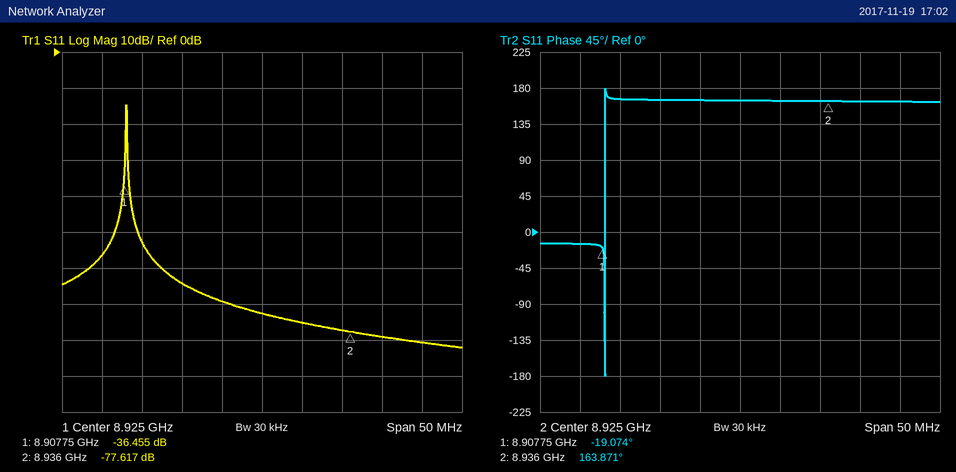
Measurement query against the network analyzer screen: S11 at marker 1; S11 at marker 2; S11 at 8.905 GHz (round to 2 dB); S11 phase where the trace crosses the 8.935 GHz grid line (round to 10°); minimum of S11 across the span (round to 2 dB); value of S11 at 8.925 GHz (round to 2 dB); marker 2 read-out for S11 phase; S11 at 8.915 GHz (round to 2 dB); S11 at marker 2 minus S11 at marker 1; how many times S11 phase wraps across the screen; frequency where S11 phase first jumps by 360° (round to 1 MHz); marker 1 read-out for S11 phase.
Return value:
-36.455 dB
-77.617 dB
-56 dB
160°
-82 dB
-72 dB
163.871°
-64 dB
-41.162 dB
1
8.908 GHz
-19.074°
